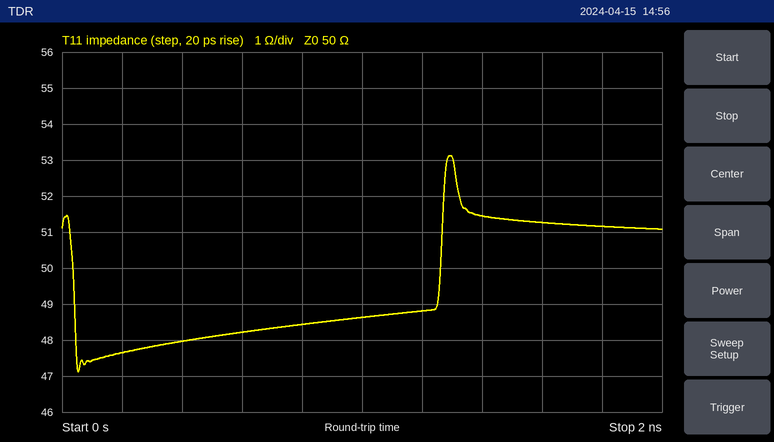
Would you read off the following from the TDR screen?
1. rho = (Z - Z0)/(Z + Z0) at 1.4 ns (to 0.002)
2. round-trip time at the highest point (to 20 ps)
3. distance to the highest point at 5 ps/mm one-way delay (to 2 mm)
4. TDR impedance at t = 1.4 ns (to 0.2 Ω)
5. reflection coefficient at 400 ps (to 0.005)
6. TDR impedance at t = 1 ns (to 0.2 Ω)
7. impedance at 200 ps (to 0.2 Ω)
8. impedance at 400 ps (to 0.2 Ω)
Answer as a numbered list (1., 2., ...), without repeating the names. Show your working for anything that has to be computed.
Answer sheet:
1. (51.4 − 50)/(51.4 + 50) ≈ +0.014
2. 1.30 ns
3. 1.30 ns / 2 / 5 ps/mm ≈ 130 mm
4. 51.4 Ω
5. (48 − 50)/(48 + 50) ≈ -0.020
6. 48.6 Ω
7. 47.6 Ω
8. 48.0 Ω
